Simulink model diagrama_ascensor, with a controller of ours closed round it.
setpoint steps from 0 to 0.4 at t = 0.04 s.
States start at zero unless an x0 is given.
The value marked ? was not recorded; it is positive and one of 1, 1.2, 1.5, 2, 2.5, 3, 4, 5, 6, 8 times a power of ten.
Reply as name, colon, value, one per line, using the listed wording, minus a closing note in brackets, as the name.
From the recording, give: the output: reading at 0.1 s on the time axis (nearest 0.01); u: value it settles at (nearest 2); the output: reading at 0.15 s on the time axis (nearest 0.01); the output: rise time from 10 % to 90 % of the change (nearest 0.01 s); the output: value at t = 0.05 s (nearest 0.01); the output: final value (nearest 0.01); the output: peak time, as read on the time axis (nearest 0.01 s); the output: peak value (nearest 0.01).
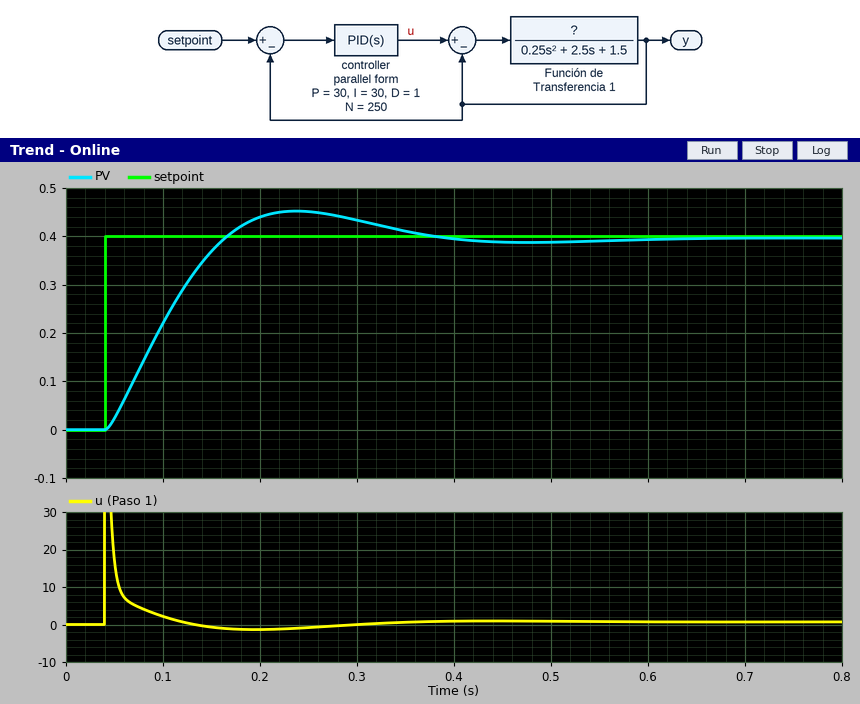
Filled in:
the output: reading at 0.1 s on the time axis: 0.22
u: value it settles at: 0
the output: reading at 0.15 s on the time axis: 0.37
the output: rise time from 10 % to 90 % of the change: 0.09 s
the output: value at t = 0.05 s: 0.02
the output: final value: 0.40
the output: peak time, as read on the time axis: 0.24 s
the output: peak value: 0.45
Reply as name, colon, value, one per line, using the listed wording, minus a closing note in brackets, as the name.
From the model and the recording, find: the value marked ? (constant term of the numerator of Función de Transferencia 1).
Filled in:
the value marked ?: 2
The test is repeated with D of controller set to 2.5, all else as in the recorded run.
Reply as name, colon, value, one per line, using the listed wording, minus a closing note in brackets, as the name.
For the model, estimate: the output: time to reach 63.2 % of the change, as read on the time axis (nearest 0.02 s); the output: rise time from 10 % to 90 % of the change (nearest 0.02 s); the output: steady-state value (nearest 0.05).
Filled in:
the output: time to reach 63.2 % of the change, as read on the time axis: 0.08 s
the output: rise time from 10 % to 90 % of the change: 0.08 s
the output: steady-state value: 0.40
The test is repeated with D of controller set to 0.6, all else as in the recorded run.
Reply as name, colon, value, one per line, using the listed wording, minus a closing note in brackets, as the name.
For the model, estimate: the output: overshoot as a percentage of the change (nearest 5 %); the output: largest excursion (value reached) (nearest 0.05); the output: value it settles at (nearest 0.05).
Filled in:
the output: overshoot as a percentage of the change: 20 %
the output: largest excursion (value reached): 0.50
the output: value it settles at: 0.40
